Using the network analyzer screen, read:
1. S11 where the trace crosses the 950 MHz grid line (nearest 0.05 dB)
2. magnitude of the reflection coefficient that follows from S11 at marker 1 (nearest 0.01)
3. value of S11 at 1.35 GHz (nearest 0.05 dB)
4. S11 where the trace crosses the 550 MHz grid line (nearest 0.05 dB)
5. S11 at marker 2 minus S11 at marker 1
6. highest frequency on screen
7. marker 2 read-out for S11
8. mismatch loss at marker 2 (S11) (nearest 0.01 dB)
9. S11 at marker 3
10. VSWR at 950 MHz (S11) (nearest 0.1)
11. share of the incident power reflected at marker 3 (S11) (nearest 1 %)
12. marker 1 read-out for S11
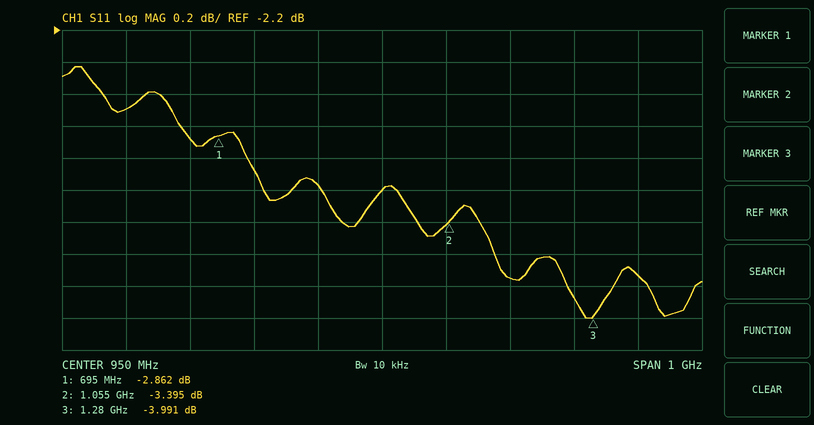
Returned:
-3.20 dB
0.72
-3.75 dB
-2.70 dB
-0.533 dB
1.45 GHz
-3.395 dB
2.66 dB
-3.991 dB
5.5
40 %
-2.862 dB
